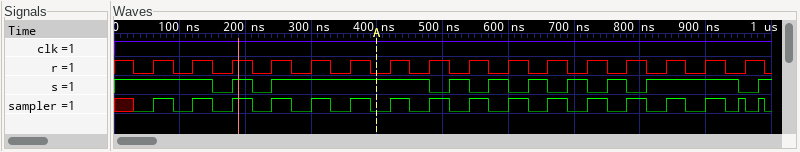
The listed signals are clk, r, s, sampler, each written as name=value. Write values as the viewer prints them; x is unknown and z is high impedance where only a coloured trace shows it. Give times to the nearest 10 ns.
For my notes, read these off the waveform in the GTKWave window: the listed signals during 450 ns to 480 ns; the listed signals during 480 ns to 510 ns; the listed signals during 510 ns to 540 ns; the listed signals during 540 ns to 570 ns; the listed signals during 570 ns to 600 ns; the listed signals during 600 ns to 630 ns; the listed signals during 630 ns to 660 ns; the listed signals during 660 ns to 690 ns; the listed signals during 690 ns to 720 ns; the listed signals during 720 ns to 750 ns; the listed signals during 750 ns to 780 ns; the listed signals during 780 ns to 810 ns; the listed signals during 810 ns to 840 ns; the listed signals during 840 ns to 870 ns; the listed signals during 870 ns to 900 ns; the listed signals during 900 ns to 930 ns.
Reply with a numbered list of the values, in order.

1. clk=1, r=0, s=1, sampler=0
2. clk=1, r=1, s=0, sampler=1
3. clk=1, r=0, s=1, sampler=0
4. clk=1, r=1, s=0, sampler=1
5. clk=1, r=0, s=1, sampler=0
6. clk=1, r=1, s=0, sampler=1
7. clk=1, r=0, s=1, sampler=0
8. clk=1, r=1, s=0, sampler=1
9. clk=1, r=0, s=1, sampler=0
10. clk=1, r=1, s=0, sampler=1
11. clk=1, r=0, s=1, sampler=0
12. clk=1, r=1, s=0, sampler=1
13. clk=1, r=0, s=1, sampler=0
14. clk=1, r=1, s=1, sampler=1
15. clk=1, r=0, s=1, sampler=0
16. clk=1, r=1, s=1, sampler=1
